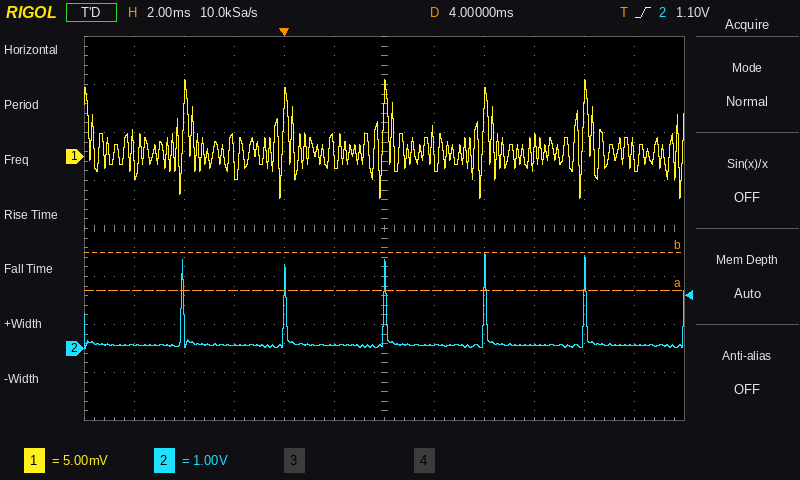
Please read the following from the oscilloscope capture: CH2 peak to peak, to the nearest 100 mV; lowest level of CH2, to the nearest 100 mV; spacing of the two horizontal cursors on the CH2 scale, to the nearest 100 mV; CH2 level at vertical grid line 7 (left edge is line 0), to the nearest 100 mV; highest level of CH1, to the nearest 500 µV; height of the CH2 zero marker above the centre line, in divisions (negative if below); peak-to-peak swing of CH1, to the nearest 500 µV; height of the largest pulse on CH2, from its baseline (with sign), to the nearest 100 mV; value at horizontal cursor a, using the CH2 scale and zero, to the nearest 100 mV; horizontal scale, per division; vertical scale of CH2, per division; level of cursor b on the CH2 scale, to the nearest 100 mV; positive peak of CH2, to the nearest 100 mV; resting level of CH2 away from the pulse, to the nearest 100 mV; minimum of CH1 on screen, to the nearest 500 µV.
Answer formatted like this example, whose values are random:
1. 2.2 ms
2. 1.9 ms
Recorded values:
1. 2.0 V
2. 0.0 V
3. 800 mV
4. 100 mV
5. 8.0 mV
6. -2.5 div
7. 12.5 mV
8. +1.9 V
9. 1.2 V
10. 2 ms
11. 1 V
12. 2.0 V
13. 2.0 V
14. 100 mV
15. -4.5 mV
